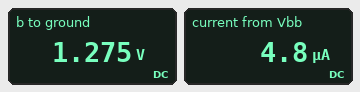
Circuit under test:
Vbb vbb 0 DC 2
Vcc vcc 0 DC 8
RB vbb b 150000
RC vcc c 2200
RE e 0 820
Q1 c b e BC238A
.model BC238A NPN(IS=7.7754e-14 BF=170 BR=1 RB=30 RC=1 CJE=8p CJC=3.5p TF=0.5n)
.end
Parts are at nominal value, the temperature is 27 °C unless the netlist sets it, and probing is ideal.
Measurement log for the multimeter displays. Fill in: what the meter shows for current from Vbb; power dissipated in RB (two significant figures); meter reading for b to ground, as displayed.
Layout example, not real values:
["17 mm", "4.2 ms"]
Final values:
["4.8 µA", "3.5 µW", "1.275 V"]
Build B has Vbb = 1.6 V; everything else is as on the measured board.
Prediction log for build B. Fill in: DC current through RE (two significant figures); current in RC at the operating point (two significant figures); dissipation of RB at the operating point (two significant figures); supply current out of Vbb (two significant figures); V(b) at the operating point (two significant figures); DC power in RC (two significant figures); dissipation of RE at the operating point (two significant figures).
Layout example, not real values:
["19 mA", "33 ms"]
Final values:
["600 µA", "590 µA", "1.8 µW", "3.5 µA", "1.1 V", "770 µW", "290 µW"]
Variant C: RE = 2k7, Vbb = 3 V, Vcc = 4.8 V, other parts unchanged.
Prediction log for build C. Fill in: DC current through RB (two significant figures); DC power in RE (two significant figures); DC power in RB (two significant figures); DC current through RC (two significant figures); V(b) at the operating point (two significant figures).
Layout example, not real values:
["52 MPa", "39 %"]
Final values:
["3.9 µA", "1.2 mW", "2.3 µW", "670 µA", "2.4 V"]
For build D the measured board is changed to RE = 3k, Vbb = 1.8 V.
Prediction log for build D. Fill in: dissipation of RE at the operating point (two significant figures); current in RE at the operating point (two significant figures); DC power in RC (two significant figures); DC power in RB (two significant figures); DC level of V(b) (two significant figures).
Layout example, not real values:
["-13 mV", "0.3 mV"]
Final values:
["300 µW", "320 µA", "220 µW", "510 nW", "1.5 V"]
